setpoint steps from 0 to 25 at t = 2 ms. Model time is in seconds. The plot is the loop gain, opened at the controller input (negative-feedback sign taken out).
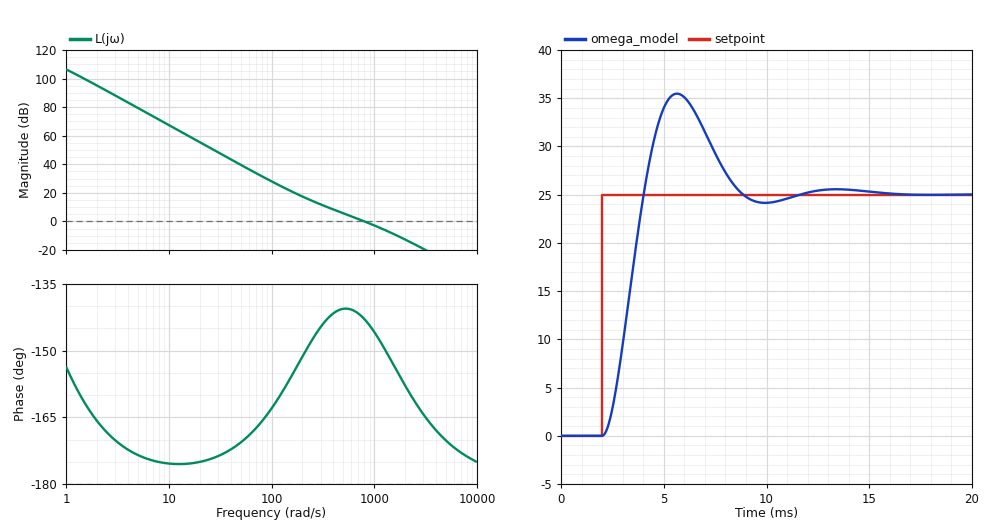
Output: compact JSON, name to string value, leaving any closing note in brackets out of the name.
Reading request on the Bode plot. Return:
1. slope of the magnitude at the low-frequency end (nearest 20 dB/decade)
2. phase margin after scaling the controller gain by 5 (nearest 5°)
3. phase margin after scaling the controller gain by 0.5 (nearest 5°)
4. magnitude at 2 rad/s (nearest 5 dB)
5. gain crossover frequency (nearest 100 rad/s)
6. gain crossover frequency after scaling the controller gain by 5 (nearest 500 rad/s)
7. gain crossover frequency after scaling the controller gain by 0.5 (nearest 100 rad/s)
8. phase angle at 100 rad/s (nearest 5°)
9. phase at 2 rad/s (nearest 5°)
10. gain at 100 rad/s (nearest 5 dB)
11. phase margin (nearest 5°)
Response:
{"slope of the magnitude at the low-frequency end": "-40 dB/decade", "phase margin after scaling the controller gain by 5": "20°", "phase margin after scaling the controller gain by 0.5": "40°", "magnitude at 2 rad/s": "95 dB", "gain crossover frequency": "800 rad/s", "gain crossover frequency after scaling the controller gain by 5": "2000 rad/s", "gain crossover frequency after scaling the controller gain by 0.5": "500 rad/s", "phase angle at 100 rad/s": "-165°", "phase at 2 rad/s": "-165°", "gain at 100 rad/s": "30 dB", "phase margin": "35°"}
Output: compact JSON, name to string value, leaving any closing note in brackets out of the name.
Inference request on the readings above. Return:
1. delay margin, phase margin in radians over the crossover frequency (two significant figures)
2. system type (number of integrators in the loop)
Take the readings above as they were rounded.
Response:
{"delay margin, phase margin in radians over the crossover frequency": "0.00076 s", "system type": "2"}
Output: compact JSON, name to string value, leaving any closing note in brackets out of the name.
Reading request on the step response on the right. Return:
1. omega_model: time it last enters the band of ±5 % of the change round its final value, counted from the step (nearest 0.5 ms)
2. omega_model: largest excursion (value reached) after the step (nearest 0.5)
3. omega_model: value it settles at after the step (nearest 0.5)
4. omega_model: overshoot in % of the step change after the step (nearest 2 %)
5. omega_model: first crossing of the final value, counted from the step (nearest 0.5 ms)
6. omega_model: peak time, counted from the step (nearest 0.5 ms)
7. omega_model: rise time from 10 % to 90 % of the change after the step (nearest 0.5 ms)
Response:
{"omega_model: time it last enters the band of ±5 % of the change round its final value, counted from the step": "6.5 ms", "omega_model: largest excursion (value reached) after the step": "35.5", "omega_model: value it settles at after the step": "25.0", "omega_model: overshoot in % of the step change after the step": "42 %", "omega_model: first crossing of the final value, counted from the step": "2.0 ms", "omega_model: peak time, counted from the step": "3.5 ms", "omega_model: rise time from 10 % to 90 % of the change after the step": "1.5 ms"}
